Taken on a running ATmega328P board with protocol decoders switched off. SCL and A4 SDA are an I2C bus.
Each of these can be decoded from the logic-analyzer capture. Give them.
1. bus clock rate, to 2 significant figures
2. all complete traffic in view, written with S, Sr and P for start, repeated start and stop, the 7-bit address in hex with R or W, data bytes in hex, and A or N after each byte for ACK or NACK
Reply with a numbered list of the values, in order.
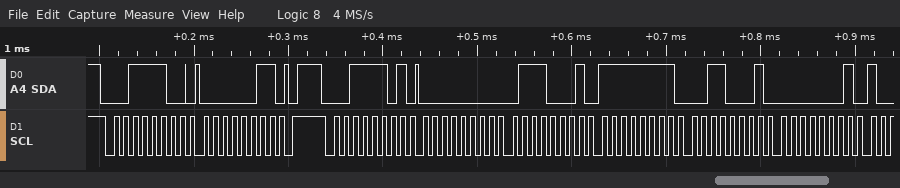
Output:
1. 100 kHz
2. S 1EW A 03 A P S 1ER A 00 A 71 A FF A 31 A 01 A
